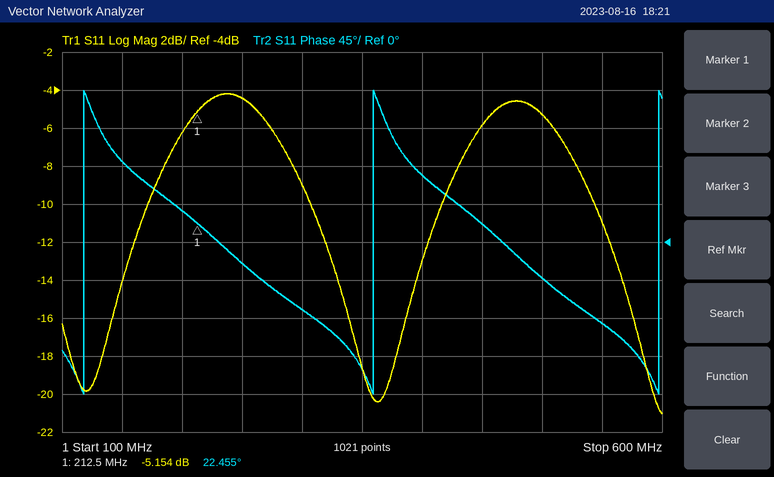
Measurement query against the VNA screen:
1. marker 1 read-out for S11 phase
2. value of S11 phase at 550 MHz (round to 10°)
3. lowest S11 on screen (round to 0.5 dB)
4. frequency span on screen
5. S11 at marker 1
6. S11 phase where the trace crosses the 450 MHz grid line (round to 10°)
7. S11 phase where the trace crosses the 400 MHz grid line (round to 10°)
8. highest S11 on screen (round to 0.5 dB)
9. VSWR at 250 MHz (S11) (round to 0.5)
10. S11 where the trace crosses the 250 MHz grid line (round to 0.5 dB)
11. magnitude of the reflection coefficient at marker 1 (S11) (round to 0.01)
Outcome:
22.455°
-100°
-21.0 dB
500 MHz
-5.154 dB
20°
80°
-4.0 dB
4.0
-4.5 dB
0.55
